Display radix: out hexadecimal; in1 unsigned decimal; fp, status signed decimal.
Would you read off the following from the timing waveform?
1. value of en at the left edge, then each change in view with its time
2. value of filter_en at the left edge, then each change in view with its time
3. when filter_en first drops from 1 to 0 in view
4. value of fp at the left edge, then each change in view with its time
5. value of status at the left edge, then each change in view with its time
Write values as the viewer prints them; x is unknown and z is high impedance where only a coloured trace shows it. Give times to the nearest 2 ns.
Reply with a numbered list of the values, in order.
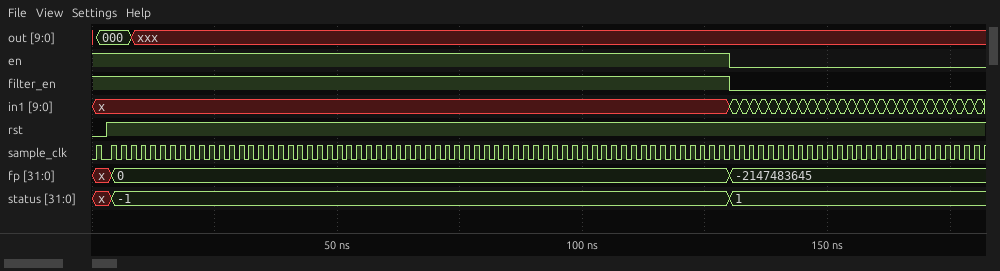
1. 1, 0 at 130 ns
2. 1, 0 at 130 ns
3. 130 ns
4. x, 0 at 4 ns, -2147483645 at 130 ns
5. x, -1 at 4 ns, 1 at 130 ns
